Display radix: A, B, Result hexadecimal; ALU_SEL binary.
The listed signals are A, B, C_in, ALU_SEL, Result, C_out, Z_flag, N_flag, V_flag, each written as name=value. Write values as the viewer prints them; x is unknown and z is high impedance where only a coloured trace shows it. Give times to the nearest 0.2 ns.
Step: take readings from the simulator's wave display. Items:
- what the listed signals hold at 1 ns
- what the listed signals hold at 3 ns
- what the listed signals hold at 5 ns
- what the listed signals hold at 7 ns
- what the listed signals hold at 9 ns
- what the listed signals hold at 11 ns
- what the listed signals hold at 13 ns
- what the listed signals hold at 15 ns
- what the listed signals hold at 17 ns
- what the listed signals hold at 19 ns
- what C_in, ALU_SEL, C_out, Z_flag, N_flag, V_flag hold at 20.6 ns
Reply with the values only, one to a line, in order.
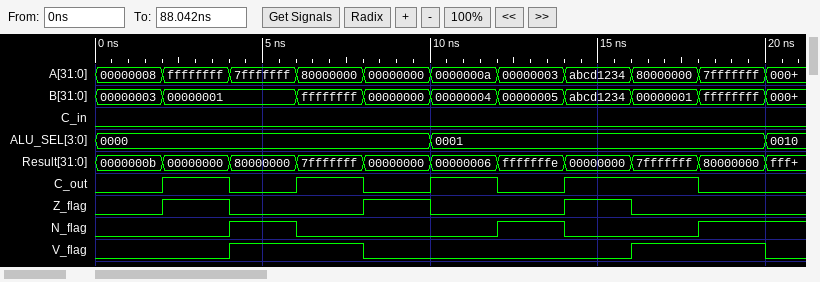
A=00000008, B=00000003, C_in=0, ALU_SEL=0000, Result=0000000b, C_out=0, Z_flag=0, N_flag=0, V_flag=0
A=ffffffff, B=00000001, C_in=0, ALU_SEL=0000, Result=00000000, C_out=1, Z_flag=1, N_flag=0, V_flag=0
A=7fffffff, B=00000001, C_in=0, ALU_SEL=0000, Result=80000000, C_out=0, Z_flag=0, N_flag=1, V_flag=1
A=80000000, B=ffffffff, C_in=0, ALU_SEL=0000, Result=7fffffff, C_out=1, Z_flag=0, N_flag=0, V_flag=1
A=00000000, B=00000000, C_in=0, ALU_SEL=0000, Result=00000000, C_out=0, Z_flag=1, N_flag=0, V_flag=0
A=0000000a, B=00000004, C_in=0, ALU_SEL=0001, Result=00000006, C_out=1, Z_flag=0, N_flag=0, V_flag=0
A=00000003, B=00000005, C_in=0, ALU_SEL=0001, Result=fffffffe, C_out=0, Z_flag=0, N_flag=1, V_flag=0
A=abcd1234, B=abcd1234, C_in=0, ALU_SEL=0001, Result=00000000, C_out=1, Z_flag=1, N_flag=0, V_flag=0
A=80000000, B=00000001, C_in=0, ALU_SEL=0001, Result=7fffffff, C_out=1, Z_flag=0, N_flag=0, V_flag=1
A=7fffffff, B=ffffffff, C_in=0, ALU_SEL=0001, Result=80000000, C_out=0, Z_flag=0, N_flag=1, V_flag=1
C_in=0, ALU_SEL=0010, C_out=0, Z_flag=0, N_flag=1, V_flag=0
